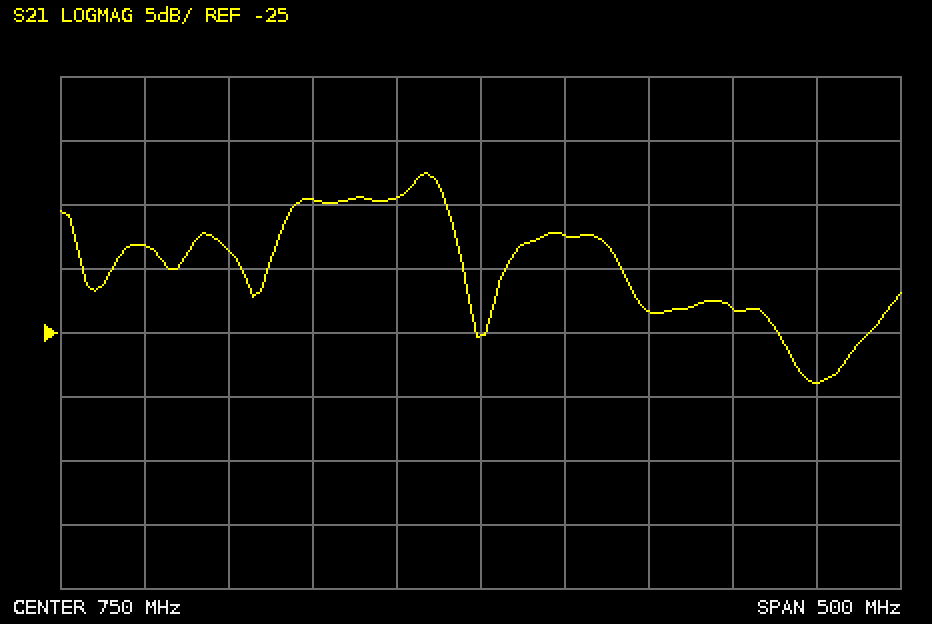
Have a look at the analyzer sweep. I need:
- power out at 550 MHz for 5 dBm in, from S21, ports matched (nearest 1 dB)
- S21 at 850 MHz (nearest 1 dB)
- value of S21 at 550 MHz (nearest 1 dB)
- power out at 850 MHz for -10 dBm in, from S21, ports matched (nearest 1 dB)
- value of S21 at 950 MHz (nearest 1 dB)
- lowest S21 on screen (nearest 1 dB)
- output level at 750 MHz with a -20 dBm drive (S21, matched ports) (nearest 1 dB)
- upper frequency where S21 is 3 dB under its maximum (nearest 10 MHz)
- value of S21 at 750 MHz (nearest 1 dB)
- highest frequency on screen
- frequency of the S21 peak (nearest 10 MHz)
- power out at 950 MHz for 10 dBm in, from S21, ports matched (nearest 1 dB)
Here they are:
-13 dBm
-23 dB
-18 dB
-33 dBm
-29 dB
-29 dB
-45 dBm
730 MHz
-25 dB
1 GHz
720 MHz
-19 dBm
